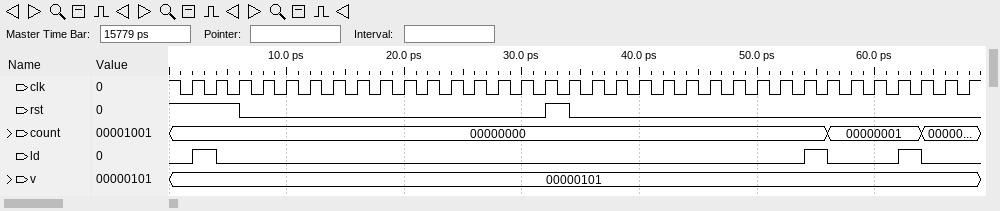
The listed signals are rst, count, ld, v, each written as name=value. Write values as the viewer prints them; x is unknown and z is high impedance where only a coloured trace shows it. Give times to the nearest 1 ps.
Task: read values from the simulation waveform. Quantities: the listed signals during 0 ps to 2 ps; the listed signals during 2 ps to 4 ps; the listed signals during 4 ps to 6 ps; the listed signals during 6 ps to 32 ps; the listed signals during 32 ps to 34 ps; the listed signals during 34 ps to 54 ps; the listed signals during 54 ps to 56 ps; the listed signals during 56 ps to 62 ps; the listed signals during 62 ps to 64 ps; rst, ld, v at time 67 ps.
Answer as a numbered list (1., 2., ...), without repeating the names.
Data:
1. rst=1, count=00000000, ld=0, v=00000101
2. rst=1, count=00000000, ld=1, v=00000101
3. rst=1, count=00000000, ld=0, v=00000101
4. rst=0, count=00000000, ld=0, v=00000101
5. rst=1, count=00000000, ld=0, v=00000101
6. rst=0, count=00000000, ld=0, v=00000101
7. rst=0, count=00000000, ld=1, v=00000101
8. rst=0, count=00000001, ld=0, v=00000101
9. rst=0, count=00000001, ld=1, v=00000101
10. rst=0, ld=0, v=00000101
